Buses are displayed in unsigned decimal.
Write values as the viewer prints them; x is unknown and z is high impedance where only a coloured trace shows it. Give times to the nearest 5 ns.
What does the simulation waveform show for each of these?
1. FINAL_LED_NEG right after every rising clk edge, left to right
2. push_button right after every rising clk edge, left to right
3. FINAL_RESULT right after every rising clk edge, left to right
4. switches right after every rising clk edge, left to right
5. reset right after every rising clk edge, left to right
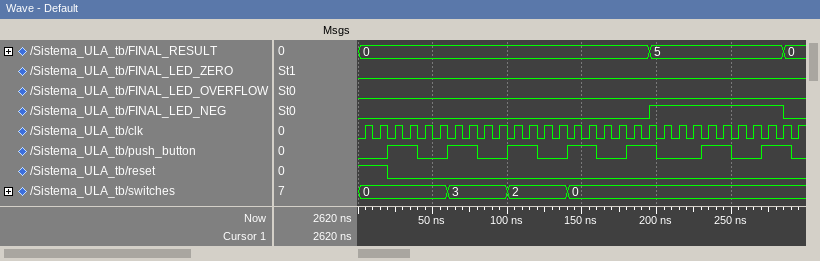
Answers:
0 0 0 0 0 0 0 0 0 0 0 0 0 0 0 0 0 0 0 1 1 1 1 1 1 1 1 1 0 0
0 0 1 1 0 0 1 1 0 0 1 1 0 0 1 1 0 0 1 1 0 0 0 1 1 0 0 1 1 0
0, 0, 0, 0, 0, 0, 0, 0, 0, 0, 0, 0, 0, 0, 0, 0, 0, 0, 0, 5, 5, 5, 5, 5, 5, 5, 5, 5, 0, 0
0, 0, 0, 0, 0, 0, 3, 3, 3, 3, 2, 2, 2, 2, 0, 0, 0, 0, 0, 0, 0, 0, 0, 0, 0, 0, 0, 0, 0, 0
1 1 0 0 0 0 0 0 0 0 0 0 0 0 0 0 0 0 0 0 0 0 0 0 0 0 0 0 0 0
